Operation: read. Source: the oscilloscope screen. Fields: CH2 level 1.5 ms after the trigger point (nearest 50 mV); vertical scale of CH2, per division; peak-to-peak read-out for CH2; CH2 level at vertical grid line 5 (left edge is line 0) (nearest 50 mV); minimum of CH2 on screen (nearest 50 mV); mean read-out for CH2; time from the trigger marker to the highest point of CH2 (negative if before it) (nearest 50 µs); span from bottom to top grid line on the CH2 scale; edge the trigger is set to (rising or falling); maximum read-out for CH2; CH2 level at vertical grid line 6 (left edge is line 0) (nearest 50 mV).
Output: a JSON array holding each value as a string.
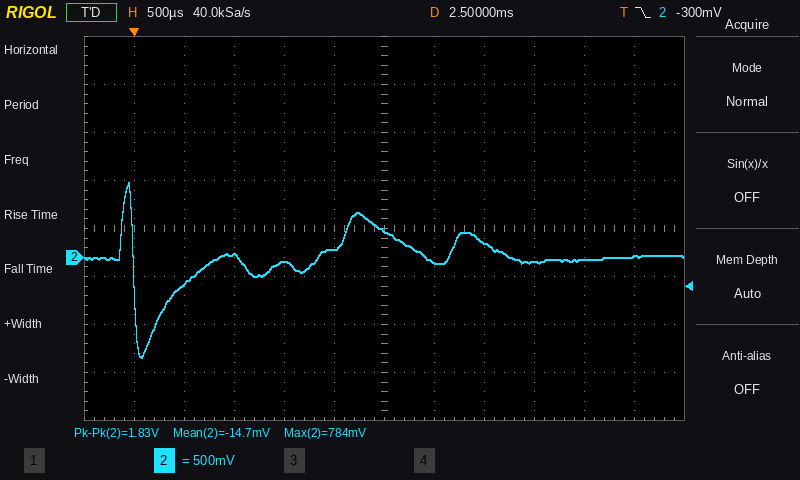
["-50 mV", "500 mV", "1.83 V", "100 mV", "-1.05 V", "-14.7 mV", "-50 µs", "4 V", "falling", "784 mV", "300 mV"]
